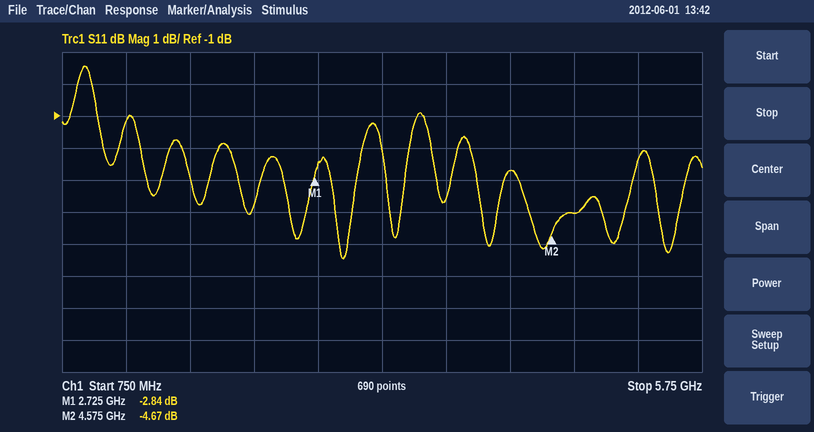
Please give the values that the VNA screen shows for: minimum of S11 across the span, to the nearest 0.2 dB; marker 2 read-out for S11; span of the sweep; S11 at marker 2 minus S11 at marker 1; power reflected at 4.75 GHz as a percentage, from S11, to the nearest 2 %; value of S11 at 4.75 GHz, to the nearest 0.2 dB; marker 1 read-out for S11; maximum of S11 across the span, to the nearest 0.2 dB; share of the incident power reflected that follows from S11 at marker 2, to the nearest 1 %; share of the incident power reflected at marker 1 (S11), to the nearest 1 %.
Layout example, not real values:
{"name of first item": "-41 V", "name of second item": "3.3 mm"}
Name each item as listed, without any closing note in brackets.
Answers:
{"minimum of S11 across the span, to the nearest 0.2 dB": "-5.4 dB", "marker 2 read-out for S11": "-4.67 dB", "span of the sweep": "5 GHz", "S11 at marker 2 minus S11 at marker 1": "-1.83 dB", "power reflected at 4.75 GHz as a percentage, from S11, to the nearest 2 %": "40 %", "value of S11 at 4.75 GHz, to the nearest 0.2 dB": "-4.0 dB", "marker 1 read-out for S11": "-2.84 dB", "maximum of S11 across the span, to the nearest 0.2 dB": "0.6 dB", "share of the incident power reflected that follows from S11 at marker 2, to the nearest 1 %": "34 %", "share of the incident power reflected at marker 1 (S11), to the nearest 1 %": "52 %"}
